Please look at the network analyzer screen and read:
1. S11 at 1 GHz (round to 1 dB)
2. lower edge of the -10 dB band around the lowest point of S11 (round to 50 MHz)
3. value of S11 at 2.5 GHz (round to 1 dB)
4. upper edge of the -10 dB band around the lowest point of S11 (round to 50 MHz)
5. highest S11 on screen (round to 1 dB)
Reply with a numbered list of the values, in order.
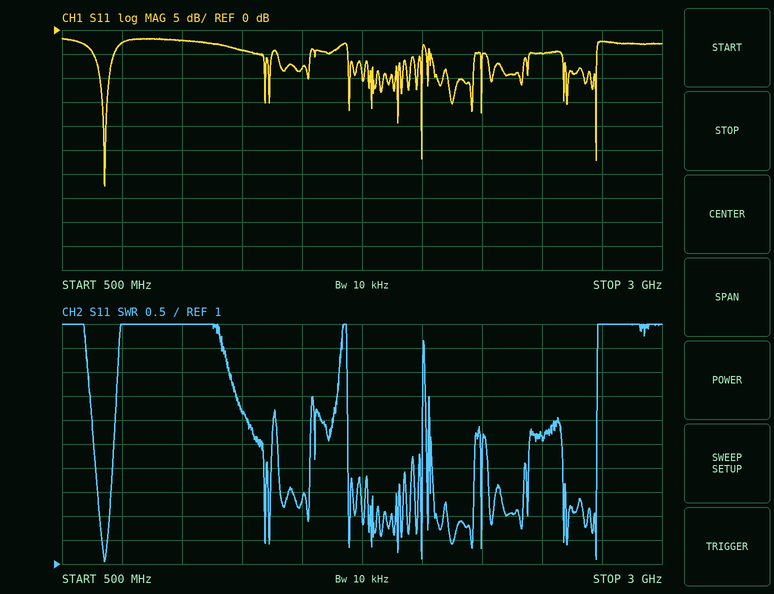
1. -2 dB
2. 650 MHz
3. -5 dB
4. 700 MHz
5. -2 dB
